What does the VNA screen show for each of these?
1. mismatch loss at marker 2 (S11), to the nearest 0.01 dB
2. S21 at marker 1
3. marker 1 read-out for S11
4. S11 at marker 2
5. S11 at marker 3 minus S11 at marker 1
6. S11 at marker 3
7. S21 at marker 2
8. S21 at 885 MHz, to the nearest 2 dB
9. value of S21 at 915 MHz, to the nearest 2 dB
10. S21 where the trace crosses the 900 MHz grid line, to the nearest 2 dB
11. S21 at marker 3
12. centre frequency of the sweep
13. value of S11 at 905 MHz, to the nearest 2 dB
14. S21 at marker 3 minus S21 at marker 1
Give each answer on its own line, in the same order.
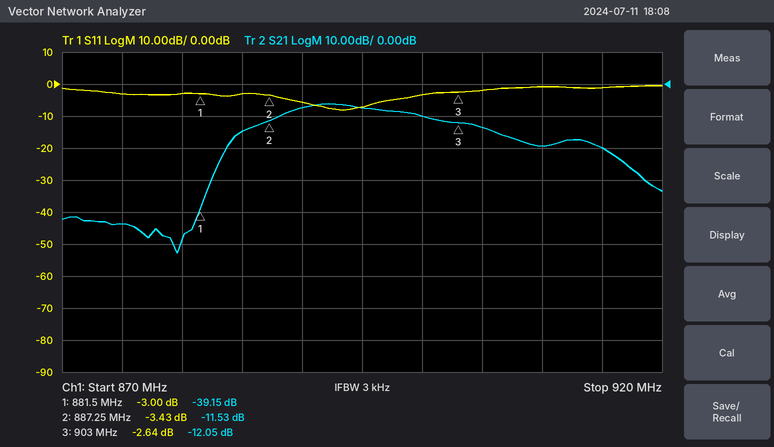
2.63 dB
-39.15 dB
-3.00 dB
-3.43 dB
0.36 dB
-2.64 dB
-11.53 dB
-14 dB
-20 dB
-10 dB
-12.05 dB
895 MHz
-2 dB
27.10 dB
